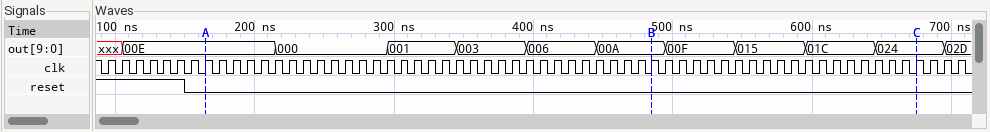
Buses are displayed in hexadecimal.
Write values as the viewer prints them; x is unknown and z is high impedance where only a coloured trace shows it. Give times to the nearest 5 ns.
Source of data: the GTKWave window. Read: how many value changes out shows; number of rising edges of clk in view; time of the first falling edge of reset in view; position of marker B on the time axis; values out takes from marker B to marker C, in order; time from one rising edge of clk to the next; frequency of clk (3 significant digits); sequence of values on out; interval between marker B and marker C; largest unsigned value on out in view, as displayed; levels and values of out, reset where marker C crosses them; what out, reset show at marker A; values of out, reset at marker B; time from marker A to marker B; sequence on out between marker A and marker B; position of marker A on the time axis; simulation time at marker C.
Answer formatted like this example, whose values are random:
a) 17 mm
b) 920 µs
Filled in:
a) 11
b) 62
c) 150 ns
d) 485 ns
e) 00A, 00F, 015, 01C, 024
f) 10 ns
g) 100 MHz
h) xxx, 00E, 000, 001, 003, 006, 00A, 00F, 015, 01C, 024, 02D
i) 190 ns
j) 02D
k) out=024, reset=0
l) out=00E, reset=0
m) out=00A, reset=0
n) 320 ns
o) 00E, 000, 001, 003, 006, 00A
p) 165 ns
q) 675 ns
